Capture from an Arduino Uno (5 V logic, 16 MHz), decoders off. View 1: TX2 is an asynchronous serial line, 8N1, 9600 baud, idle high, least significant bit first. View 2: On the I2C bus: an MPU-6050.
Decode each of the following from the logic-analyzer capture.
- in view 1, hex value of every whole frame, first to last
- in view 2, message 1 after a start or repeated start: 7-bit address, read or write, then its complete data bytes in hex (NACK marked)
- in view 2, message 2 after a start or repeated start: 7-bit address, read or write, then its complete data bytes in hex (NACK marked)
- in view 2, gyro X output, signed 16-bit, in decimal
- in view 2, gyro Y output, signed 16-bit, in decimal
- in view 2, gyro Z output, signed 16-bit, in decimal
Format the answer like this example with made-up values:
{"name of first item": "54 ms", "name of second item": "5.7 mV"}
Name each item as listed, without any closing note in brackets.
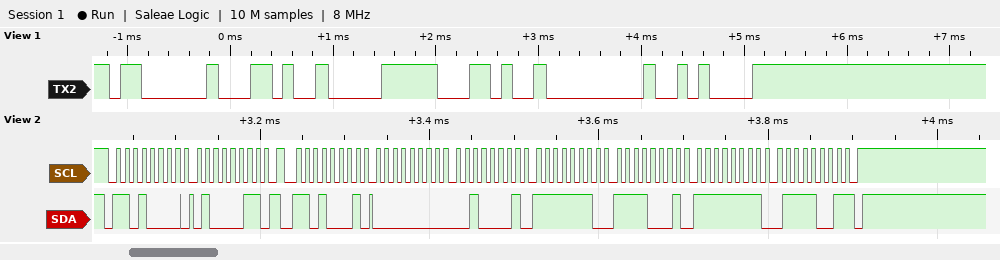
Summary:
{"in view 1, hex value of every whole frame, first to last": "03 2C F0 2C 00 0A", "in view 2, message 1 after a start or repeated start: 7-bit address, read or write, then its complete data bytes in hex": "0x68 write: 43", "in view 2, message 2 after a start or repeated start: 7-bit address, read or write, then its complete data bytes in hex": "0x68 read: 00 21 FE F1 FF 79 NACK", "in view 2, gyro X output, signed 16-bit, in decimal": "33", "in view 2, gyro Y output, signed 16-bit, in decimal": "-271", "in view 2, gyro Z output, signed 16-bit, in decimal": "-135"}
